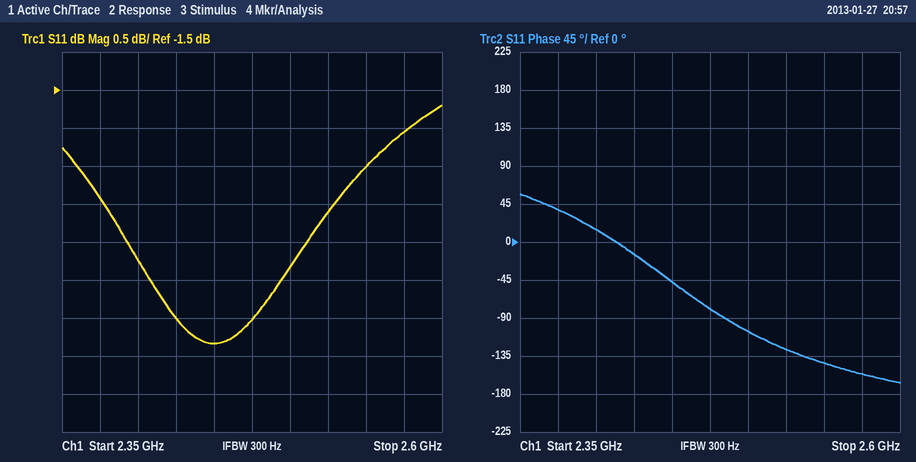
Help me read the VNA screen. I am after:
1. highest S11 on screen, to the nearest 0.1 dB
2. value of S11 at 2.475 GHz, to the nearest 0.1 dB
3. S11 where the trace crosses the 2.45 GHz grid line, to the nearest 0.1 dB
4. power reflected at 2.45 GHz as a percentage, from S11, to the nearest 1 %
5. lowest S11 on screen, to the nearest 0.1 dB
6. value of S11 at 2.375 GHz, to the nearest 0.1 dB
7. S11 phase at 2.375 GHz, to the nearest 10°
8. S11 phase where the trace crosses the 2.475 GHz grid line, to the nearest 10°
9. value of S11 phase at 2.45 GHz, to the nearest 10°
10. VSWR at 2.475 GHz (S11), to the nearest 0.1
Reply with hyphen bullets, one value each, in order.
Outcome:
- -1.7 dB
- -4.5 dB
- -4.8 dB
- 33 %
- -4.8 dB
- -2.9 dB
- 40°
- -80°
- -50°
- 3.9
